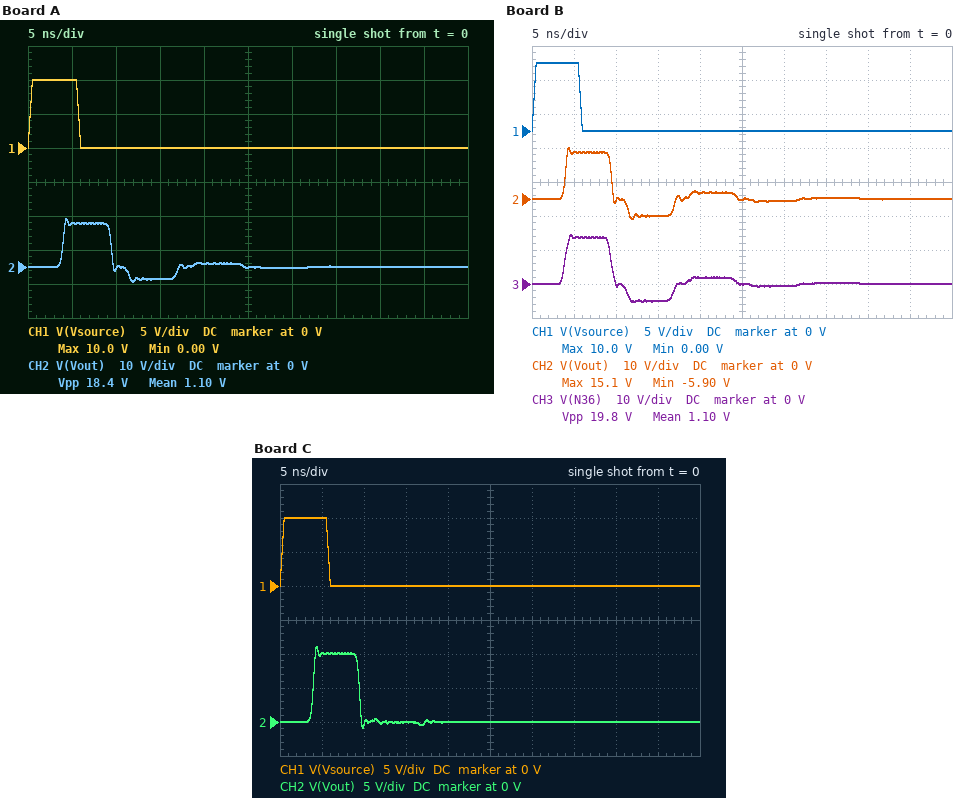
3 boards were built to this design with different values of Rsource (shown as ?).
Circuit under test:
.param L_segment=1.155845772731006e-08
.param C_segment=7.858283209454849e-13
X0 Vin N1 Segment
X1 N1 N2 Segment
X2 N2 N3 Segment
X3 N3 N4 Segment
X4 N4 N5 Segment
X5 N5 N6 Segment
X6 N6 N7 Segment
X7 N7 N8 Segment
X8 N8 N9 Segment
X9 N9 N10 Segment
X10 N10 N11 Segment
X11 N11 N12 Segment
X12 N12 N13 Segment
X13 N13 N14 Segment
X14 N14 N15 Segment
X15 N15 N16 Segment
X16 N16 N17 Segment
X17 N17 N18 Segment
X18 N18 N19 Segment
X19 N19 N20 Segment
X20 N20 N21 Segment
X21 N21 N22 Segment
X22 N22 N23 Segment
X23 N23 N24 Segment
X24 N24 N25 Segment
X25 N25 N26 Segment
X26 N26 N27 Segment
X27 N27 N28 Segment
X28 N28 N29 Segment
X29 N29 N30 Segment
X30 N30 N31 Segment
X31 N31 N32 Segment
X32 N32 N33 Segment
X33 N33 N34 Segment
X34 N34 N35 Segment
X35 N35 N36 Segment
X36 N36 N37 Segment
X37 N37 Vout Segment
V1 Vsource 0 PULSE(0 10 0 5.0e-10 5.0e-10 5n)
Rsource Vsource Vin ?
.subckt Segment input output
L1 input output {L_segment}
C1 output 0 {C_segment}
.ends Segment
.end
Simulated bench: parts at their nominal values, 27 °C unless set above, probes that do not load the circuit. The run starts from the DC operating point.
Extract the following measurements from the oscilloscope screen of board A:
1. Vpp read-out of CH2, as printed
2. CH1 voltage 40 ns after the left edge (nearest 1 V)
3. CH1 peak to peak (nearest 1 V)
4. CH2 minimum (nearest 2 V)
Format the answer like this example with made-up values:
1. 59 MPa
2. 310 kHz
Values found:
1. 18.4 V
2. 0 V
3. 10 V
4. -4 V
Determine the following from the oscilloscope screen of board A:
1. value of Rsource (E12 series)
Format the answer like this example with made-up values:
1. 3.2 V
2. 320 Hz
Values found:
1. 68 Ω
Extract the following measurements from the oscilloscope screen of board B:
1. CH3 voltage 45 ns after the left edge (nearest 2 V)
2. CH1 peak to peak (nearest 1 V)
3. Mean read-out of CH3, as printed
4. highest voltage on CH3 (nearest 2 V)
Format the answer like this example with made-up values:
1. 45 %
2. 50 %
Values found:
1. 0 V
2. 10 V
3. 1.10 V
4. 14 V
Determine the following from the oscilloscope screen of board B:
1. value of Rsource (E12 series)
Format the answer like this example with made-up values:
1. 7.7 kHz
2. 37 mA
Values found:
1. 56 Ω
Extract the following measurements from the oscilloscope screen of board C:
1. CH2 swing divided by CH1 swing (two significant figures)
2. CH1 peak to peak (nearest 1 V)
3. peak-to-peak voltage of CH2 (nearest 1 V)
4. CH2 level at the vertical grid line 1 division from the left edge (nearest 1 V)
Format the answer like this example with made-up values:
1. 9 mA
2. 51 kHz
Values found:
1. 1.2
2. 10 V
3. 12 V
4. 10 V
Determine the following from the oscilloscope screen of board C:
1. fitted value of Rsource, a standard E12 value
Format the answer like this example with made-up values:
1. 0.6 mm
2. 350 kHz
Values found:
1. 120 Ω
